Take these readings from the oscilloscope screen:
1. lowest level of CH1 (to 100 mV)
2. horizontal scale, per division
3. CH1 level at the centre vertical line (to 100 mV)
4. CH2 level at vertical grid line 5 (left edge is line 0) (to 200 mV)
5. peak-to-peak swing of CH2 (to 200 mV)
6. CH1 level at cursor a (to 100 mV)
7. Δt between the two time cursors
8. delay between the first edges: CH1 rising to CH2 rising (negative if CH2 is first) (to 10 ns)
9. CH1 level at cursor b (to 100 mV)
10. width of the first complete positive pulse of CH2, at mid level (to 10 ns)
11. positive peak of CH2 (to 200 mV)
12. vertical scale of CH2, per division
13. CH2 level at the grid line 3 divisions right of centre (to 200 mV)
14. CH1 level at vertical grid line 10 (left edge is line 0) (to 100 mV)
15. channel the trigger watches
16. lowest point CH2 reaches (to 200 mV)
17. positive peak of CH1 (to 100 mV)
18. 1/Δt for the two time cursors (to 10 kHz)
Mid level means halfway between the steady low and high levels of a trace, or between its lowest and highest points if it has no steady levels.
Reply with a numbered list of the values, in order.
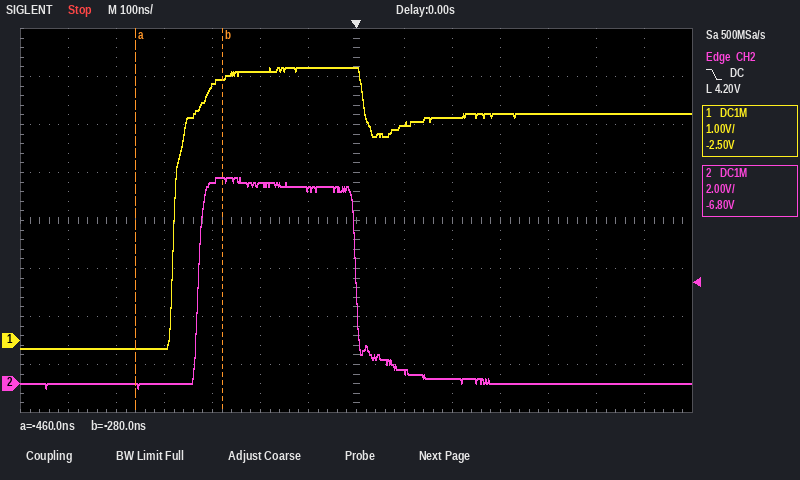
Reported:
1. -200 mV
2. 100 ns
3. 5.7 V
4. 8.4 V
5. 8.8 V
6. -200 mV
7. 180 ns
8. +50 ns
9. 5.5 V
10. 330 ns
11. 8.6 V
12. 2 V
13. 0.0 V
14. 4.7 V
15. CH2
16. -200 mV
17. 5.7 V
18. 5.56 MHz
